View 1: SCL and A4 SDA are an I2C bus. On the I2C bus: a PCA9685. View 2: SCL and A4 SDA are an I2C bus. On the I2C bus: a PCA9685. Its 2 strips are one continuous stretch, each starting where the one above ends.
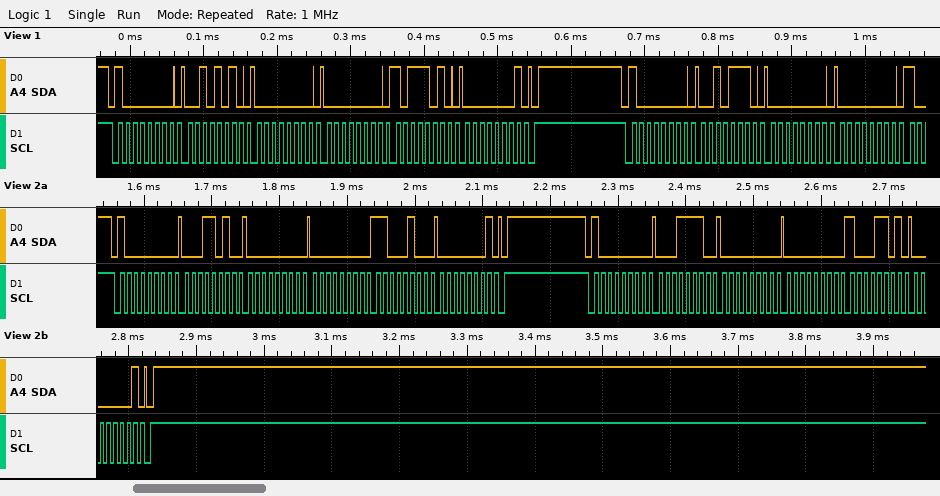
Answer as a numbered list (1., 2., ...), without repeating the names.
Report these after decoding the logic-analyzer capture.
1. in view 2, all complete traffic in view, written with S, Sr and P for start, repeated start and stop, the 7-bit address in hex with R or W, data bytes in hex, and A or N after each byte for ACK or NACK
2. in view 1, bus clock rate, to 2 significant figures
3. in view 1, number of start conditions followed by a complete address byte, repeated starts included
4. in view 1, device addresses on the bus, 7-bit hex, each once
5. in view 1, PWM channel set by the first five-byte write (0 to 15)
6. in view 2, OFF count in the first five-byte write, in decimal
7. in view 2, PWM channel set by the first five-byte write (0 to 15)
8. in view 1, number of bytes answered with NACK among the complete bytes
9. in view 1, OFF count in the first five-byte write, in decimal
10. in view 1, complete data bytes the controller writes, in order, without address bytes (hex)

1. S 40W A 1A A 00 A 00 A C4 A 01 A P S 40W A 1E A 00 A 00 A 8D A 01 A P
2. 100 kHz
3. 2
4. 0x40
5. 9
6. 452
7. 5
8. 0
9. 442
10. 2A 00 00 BA 01 2E 00 00
